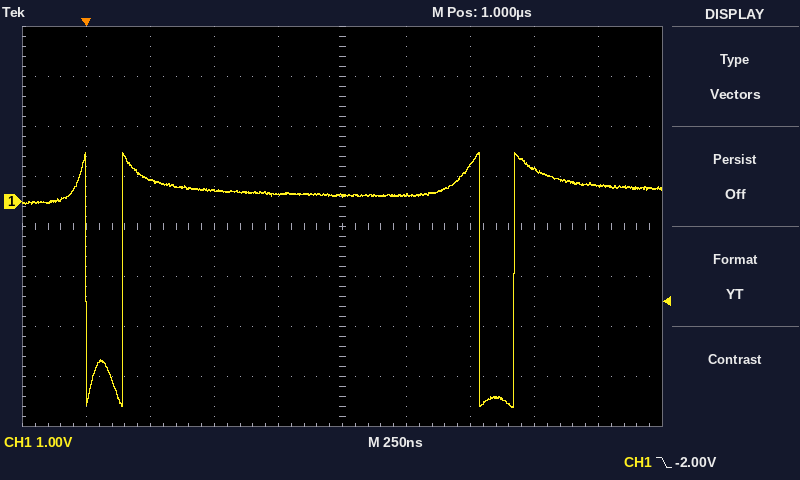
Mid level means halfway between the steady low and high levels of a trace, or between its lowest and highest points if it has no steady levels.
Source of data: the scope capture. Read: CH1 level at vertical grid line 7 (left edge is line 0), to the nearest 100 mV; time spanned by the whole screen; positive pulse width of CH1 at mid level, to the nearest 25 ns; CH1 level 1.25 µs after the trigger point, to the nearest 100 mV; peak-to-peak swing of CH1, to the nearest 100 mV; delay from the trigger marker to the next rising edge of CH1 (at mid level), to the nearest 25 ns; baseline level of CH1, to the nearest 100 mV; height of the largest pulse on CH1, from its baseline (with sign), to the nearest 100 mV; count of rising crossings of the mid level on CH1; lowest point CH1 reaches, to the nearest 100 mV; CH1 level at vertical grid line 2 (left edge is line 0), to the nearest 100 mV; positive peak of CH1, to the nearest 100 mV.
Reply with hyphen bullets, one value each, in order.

- 700 mV
- 2.5 µs
- 1.400 µs
- 100 mV
- 5.1 V
- 150 ns
- 200 mV
- -4.3 V
- 2
- -4.1 V
- 400 mV
- 1.0 V
